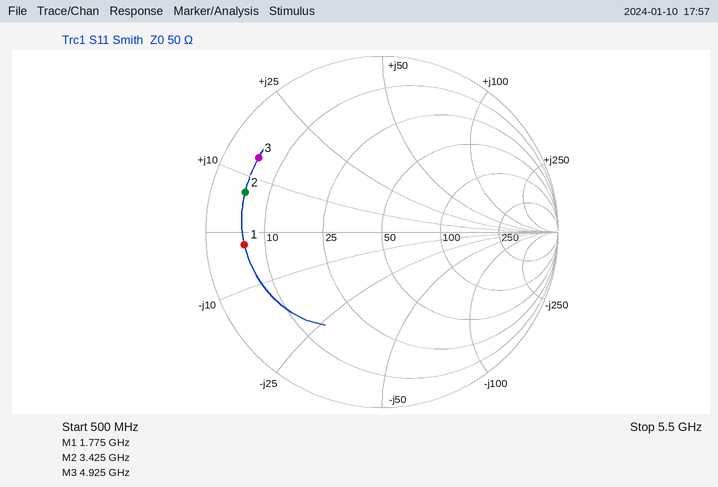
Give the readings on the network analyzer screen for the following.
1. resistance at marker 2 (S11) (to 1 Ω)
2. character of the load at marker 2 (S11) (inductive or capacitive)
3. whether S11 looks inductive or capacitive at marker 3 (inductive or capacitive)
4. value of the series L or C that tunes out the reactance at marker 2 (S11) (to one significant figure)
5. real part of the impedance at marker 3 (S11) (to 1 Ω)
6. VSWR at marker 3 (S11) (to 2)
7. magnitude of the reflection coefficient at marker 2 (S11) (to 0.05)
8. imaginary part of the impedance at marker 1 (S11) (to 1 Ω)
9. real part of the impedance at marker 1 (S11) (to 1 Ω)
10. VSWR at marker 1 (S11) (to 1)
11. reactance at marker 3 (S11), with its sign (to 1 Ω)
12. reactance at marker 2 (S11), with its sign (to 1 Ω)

5 Ω
inductive
inductive
7 pF
5 Ω
10
0.80
-2 Ω
6 Ω
8
+14 Ω
+7 Ω
